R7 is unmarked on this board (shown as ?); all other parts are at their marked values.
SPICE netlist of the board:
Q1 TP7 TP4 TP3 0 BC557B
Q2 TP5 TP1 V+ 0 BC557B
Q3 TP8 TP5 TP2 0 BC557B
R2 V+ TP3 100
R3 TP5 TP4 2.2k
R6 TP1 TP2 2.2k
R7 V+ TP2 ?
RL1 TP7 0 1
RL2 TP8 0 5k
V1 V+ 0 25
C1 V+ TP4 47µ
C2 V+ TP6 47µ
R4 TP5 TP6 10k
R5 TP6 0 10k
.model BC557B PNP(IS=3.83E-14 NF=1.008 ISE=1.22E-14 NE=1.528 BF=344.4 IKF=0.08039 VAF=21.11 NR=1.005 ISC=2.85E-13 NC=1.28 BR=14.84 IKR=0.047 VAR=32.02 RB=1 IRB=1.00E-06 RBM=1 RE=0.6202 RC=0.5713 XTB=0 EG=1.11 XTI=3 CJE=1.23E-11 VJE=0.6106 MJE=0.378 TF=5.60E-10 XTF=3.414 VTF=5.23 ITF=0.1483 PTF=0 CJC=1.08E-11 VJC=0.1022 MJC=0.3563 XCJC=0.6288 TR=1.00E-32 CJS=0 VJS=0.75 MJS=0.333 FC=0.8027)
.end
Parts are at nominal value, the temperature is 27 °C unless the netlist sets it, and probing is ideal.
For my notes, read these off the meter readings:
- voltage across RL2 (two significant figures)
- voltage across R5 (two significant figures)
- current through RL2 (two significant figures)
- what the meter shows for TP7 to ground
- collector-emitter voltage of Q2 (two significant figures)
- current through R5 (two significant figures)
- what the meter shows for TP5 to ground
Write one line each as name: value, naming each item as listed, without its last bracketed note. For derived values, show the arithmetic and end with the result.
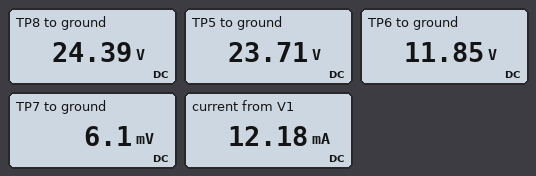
voltage across RL2: 24.39 V = 24 V
voltage across R5: 11.85 V = 12 V
current through RL2: (24.39 V) / 5 kΩ = 4.9 mA
what the meter shows for TP7 to ground: 6.1 mV
collector-emitter voltage of Q2: 23.71 V - 25 V = -1.3 V
current through R5: (11.85 V) / 10 kΩ = 1.2 mA
what the meter shows for TP5 to ground: 23.71 V
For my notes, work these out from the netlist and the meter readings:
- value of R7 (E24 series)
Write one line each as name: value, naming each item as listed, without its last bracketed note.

value of R7: 100 Ω
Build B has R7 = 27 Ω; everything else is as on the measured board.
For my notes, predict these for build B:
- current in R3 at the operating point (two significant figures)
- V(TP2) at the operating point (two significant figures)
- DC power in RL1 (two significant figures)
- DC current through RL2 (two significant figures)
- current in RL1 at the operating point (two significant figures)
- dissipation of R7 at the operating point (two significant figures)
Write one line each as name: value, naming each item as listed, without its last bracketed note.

current in R3 at the operating point: 3.4 µA
V(TP2) at the operating point: 25 V
DC power in RL1: 5.7 µW
DC current through RL2: 5.0 mA
current in RL1 at the operating point: 2.4 mA
dissipation of R7 at the operating point: 1.0 mW
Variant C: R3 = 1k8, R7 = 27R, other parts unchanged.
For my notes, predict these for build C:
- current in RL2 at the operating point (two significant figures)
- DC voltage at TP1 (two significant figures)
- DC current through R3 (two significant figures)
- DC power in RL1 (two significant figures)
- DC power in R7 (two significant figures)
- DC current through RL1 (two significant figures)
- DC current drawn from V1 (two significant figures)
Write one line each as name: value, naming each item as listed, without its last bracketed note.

current in RL2 at the operating point: 5.0 mA
DC voltage at TP1: 25 V
DC current through R3: 3.4 µA
DC power in RL1: 5.7 µW
DC power in R7: 1.0 mW
DC current through RL1: 2.4 mA
DC current drawn from V1: 8.6 mA
